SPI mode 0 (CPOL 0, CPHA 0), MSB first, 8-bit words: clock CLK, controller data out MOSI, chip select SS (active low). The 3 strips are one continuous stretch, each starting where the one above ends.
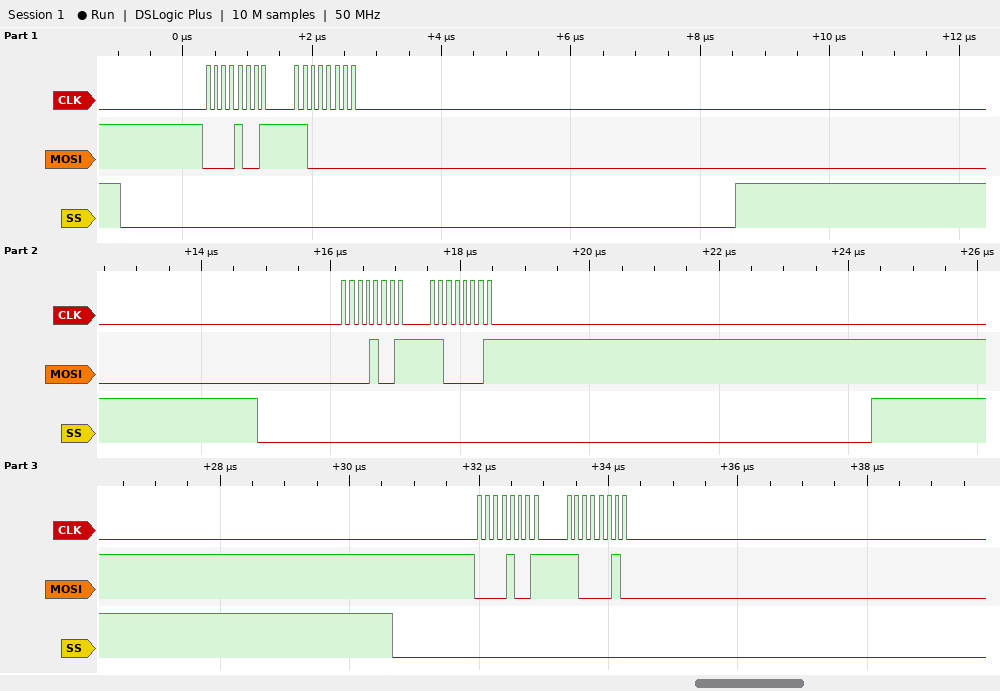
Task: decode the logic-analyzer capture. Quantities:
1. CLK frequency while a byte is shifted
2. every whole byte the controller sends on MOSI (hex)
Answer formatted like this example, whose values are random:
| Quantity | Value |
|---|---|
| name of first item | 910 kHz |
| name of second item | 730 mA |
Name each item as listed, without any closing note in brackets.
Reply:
| Quantity | Value |
|---|---|
| CLK frequency while a byte is shifted | 8 MHz |
| every whole byte the controller sends on MOSI | 09 C0 09 C1 09 C2 |
